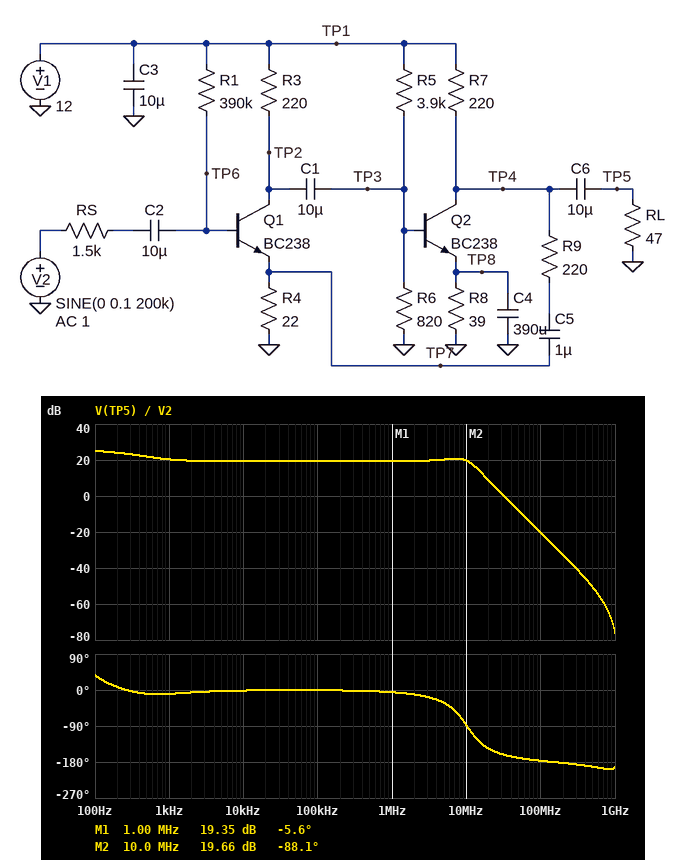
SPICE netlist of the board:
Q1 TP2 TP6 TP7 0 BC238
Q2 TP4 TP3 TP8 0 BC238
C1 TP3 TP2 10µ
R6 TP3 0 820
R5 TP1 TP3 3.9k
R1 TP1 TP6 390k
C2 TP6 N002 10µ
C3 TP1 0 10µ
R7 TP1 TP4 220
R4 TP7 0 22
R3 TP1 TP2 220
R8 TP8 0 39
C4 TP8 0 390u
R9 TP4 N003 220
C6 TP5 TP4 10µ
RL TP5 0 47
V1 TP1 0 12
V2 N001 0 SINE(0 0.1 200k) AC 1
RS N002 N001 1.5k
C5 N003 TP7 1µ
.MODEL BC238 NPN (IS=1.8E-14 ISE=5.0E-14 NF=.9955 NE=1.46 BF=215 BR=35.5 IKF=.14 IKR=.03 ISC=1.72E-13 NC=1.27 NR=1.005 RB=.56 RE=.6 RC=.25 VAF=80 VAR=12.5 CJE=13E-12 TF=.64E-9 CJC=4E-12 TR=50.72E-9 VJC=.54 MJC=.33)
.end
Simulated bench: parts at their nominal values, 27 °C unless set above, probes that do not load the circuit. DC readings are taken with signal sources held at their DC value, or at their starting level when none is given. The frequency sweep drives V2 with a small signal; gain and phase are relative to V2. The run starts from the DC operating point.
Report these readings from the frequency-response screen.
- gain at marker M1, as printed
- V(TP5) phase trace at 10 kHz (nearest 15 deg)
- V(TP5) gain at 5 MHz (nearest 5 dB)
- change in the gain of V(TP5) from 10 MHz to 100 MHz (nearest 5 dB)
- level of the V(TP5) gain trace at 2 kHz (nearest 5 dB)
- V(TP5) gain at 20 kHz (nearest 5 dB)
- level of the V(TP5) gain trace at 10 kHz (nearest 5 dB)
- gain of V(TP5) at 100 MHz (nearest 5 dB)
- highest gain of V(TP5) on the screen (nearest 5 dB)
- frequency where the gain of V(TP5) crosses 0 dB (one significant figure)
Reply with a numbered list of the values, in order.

1. 19.35 dB
2. 0 deg
3. 20 dB
4. -40 dB
5. 20 dB
6. 20 dB
7. 20 dB
8. -20 dB
9. 25 dB
10. 30 MHz
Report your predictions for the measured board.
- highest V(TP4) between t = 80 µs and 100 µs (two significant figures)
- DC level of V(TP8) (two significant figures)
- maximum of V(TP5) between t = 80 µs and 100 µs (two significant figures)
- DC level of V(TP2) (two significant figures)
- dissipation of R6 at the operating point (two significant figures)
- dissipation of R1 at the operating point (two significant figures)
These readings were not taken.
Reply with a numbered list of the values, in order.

1. 6.1 V
2. 1.2 V
3. 880 mV
4. 11 V
5. 4.7 mW
6. 320 µW
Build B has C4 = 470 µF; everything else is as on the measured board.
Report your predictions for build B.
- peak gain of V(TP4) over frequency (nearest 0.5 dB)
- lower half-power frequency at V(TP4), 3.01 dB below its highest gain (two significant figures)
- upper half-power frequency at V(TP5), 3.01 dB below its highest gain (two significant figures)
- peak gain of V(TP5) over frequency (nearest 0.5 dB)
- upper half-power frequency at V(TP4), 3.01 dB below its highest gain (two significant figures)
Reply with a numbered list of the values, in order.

1. 41.0 dB
2. 33 Hz
3. 380 Hz
4. 25.5 dB
5. 83 Hz
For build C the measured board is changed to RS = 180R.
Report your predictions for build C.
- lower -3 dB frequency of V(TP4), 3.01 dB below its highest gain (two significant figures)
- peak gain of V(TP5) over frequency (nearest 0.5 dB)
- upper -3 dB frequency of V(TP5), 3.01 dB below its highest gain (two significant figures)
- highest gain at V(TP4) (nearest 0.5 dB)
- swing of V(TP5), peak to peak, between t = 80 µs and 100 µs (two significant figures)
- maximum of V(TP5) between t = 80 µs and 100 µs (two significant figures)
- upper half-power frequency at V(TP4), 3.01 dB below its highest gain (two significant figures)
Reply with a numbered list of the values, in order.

1. 33 Hz
2. 26.5 dB
3. 330 Hz
4. 42.0 dB
5. 1.9 V
6. 910 mV
7. 81 Hz
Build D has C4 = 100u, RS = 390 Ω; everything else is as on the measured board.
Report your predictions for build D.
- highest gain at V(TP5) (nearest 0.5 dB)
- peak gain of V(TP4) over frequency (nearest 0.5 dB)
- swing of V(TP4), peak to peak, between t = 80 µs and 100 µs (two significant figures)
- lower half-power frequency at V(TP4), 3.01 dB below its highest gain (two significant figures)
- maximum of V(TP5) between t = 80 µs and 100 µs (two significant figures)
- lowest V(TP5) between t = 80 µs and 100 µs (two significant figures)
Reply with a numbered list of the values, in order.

1. 23.5 dB
2. 31.5 dB
3. 1.9 V
4. 27 Hz
5. 910 mV
6. -950 mV
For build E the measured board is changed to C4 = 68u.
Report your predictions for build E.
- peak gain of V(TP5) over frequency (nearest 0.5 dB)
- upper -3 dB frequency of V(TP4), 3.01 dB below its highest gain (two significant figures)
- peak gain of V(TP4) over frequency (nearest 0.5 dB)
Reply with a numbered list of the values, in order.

1. 22.5 dB
2. 430 Hz
3. 27.5 dB
